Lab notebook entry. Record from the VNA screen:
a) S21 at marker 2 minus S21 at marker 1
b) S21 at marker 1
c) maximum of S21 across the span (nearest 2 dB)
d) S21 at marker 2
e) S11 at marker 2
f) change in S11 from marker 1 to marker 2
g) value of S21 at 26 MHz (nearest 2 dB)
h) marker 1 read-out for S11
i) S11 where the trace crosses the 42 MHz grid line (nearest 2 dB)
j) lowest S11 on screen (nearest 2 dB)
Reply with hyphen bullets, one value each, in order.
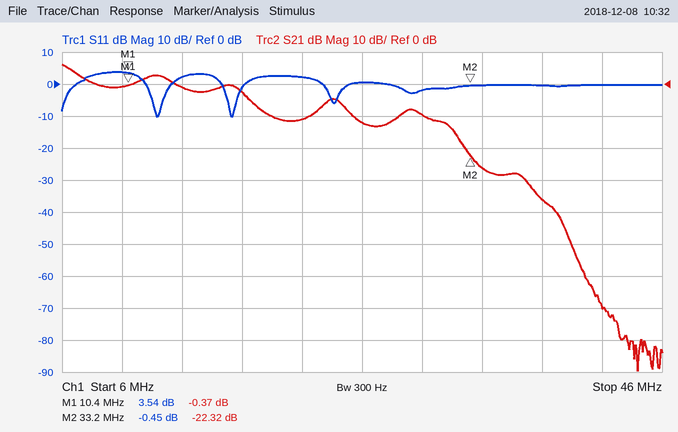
- -21.95 dB
- -0.37 dB
- 6 dB
- -22.32 dB
- -0.45 dB
- -3.99 dB
- -12 dB
- 3.54 dB
- 0 dB
- -10 dB
